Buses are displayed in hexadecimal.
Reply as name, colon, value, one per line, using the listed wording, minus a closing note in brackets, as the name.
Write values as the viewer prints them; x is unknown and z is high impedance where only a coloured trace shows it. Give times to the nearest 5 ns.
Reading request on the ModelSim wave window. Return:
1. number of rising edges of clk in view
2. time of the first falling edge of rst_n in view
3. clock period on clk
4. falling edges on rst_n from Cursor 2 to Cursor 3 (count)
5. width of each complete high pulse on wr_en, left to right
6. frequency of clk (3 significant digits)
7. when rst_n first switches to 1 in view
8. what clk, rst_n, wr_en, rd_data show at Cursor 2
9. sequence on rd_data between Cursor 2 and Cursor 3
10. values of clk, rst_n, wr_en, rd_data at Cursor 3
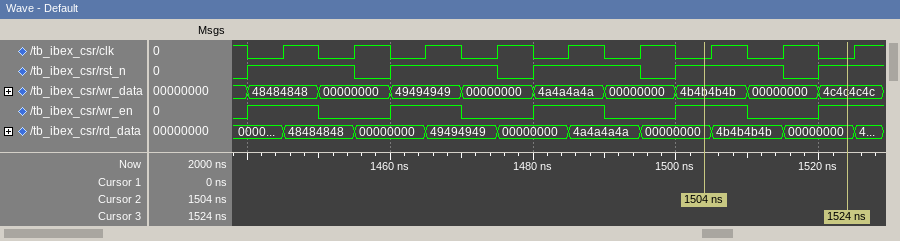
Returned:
number of rising edges of clk in view: 9
time of the first falling edge of rst_n in view: 1455 ns
clock period on clk: 10 ns
falling edges on rst_n from Cursor 2 to Cursor 3: 1
width of each complete high pulse on wr_en, left to right: 10 ns, 10 ns, 10 ns, 10 ns
frequency of clk: 100 MHz
when rst_n first switches to 1 in view: 1440 ns
what clk, rst_n, wr_en, rd_data show at Cursor 2: clk=0, rst_n=1, wr_en=1, rd_data=00000000
sequence on rd_data between Cursor 2 and Cursor 3: 00000000, 4b4b4b4b, 00000000
values of clk, rst_n, wr_en, rd_data at Cursor 3: clk=0, rst_n=1, wr_en=1, rd_data=00000000
